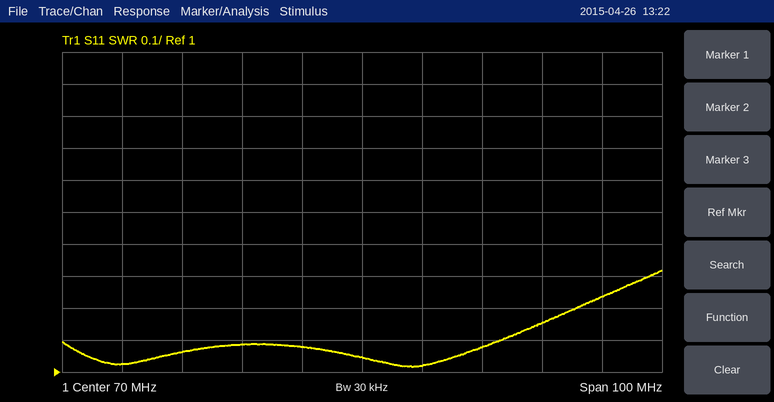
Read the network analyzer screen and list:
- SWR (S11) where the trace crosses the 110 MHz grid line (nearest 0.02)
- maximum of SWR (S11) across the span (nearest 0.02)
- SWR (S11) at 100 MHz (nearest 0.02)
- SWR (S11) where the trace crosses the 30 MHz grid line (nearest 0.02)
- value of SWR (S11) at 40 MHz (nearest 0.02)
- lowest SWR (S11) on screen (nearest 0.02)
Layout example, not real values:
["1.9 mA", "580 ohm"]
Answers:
["1.24", "1.32", "1.16", "1.02", "1.06", "1.02"]
